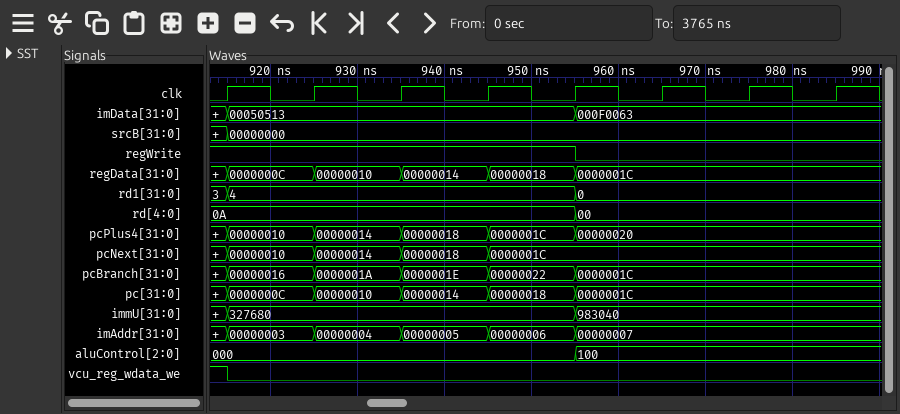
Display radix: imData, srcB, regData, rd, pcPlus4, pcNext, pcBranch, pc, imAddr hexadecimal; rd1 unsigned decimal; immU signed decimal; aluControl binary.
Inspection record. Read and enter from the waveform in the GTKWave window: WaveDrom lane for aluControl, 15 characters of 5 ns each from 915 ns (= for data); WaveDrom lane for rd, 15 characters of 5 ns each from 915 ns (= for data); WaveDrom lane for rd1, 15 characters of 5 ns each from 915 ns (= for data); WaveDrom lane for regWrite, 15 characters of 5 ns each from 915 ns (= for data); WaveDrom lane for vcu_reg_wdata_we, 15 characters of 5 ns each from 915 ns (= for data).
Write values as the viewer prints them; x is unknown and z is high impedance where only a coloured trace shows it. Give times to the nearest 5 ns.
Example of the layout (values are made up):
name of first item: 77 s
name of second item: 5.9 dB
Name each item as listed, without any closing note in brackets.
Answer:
WaveDrom lane for aluControl, 15 characters of 5 ns each from 915 ns: {name: 'aluControl', wave: '=.......=......', data: '000 100'}
WaveDrom lane for rd, 15 characters of 5 ns each from 915 ns: {name: 'rd', wave: '=.......=......', data: '0A 00'}
WaveDrom lane for rd1, 15 characters of 5 ns each from 915 ns: {name: 'rd1', wave: '=.......=......', data: '4 0'}
WaveDrom lane for regWrite, 15 characters of 5 ns each from 915 ns: {name: 'regWrite', wave: '1.......0......'}
WaveDrom lane for vcu_reg_wdata_we, 15 characters of 5 ns each from 915 ns: {name: 'vcu_reg_wdata_we', wave: '0..............'}
